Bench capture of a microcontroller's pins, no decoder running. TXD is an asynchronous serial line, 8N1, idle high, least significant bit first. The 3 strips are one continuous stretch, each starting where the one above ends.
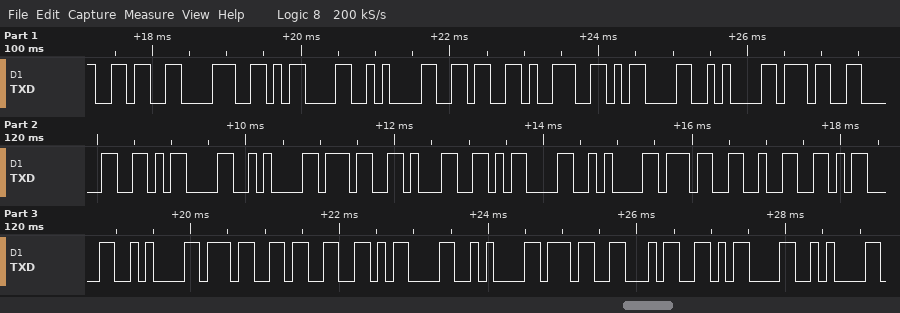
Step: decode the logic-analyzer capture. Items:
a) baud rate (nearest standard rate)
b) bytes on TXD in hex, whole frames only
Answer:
9600 baud
36 38 0D 0A 36 39 0D 0A 37 30 0D 0A 37 31 0D 0A 37 32 0D 0A 37 33 0D 0A 37 34 0D 0A
